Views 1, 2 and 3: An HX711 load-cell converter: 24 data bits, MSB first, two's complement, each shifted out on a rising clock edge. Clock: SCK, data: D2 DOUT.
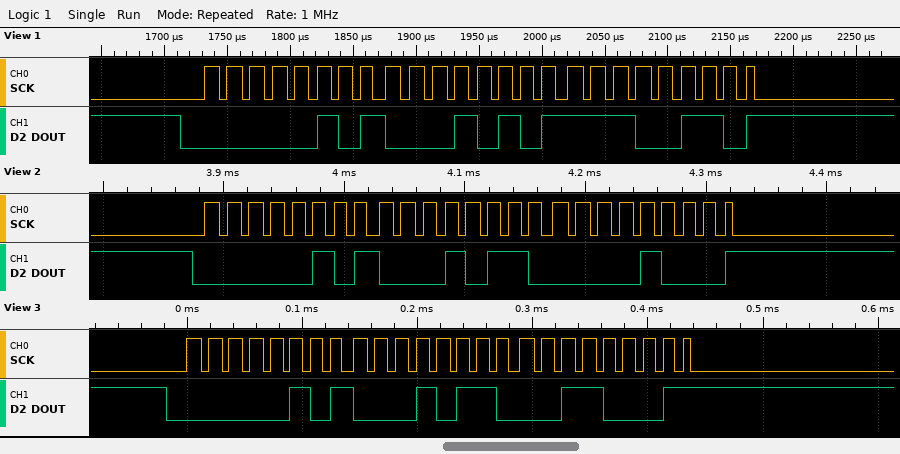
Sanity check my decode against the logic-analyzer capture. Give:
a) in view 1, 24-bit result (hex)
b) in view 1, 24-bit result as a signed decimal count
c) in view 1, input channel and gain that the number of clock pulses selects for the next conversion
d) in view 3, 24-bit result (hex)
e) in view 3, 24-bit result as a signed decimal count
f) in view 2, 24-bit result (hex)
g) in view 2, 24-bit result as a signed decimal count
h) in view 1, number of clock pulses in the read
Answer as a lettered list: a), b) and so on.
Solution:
a) 0x0515E6
b) 333286
c) channel A, gain 128
d) 0x051631
e) 333361
f) 0x051608
g) 333320
h) 25
